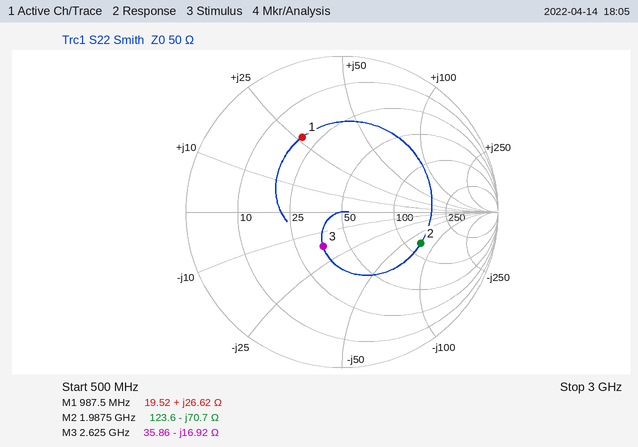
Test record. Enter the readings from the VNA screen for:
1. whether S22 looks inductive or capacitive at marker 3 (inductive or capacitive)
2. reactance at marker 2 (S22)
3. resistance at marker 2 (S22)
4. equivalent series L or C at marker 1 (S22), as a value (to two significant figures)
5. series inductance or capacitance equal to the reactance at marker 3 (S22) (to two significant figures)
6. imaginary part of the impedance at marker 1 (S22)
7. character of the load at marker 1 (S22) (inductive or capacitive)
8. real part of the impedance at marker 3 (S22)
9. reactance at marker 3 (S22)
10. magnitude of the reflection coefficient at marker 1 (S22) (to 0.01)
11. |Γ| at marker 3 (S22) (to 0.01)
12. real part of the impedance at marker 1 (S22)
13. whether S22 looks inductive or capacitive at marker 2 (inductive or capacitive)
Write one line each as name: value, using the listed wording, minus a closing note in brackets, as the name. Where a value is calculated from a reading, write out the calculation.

whether S22 looks inductive or capacitive at marker 3: capacitive
reactance at marker 2: -70.7 Ω
resistance at marker 2: 123.6 Ω
equivalent series L or C at marker 1 (S22), as a value: L = 26.62 Ω/(2π × 987.5 MHz) ≈ 4.3 nH
series inductance or capacitance equal to the reactance at marker 3 (S22): C = 1/(2π × 2.625 GHz × 16.92 Ω) ≈ 3.6 pF
imaginary part of the impedance at marker 1: +26.62 Ω
character of the load at marker 1 (S22): inductive
real part of the impedance at marker 3: 35.86 Ω
reactance at marker 3: -16.92 Ω
magnitude of the reflection coefficient at marker 1 (S22): 0.54
|Γ| at marker 3 (S22): 0.25
real part of the impedance at marker 1: 19.52 Ω
whether S22 looks inductive or capacitive at marker 2: capacitive
